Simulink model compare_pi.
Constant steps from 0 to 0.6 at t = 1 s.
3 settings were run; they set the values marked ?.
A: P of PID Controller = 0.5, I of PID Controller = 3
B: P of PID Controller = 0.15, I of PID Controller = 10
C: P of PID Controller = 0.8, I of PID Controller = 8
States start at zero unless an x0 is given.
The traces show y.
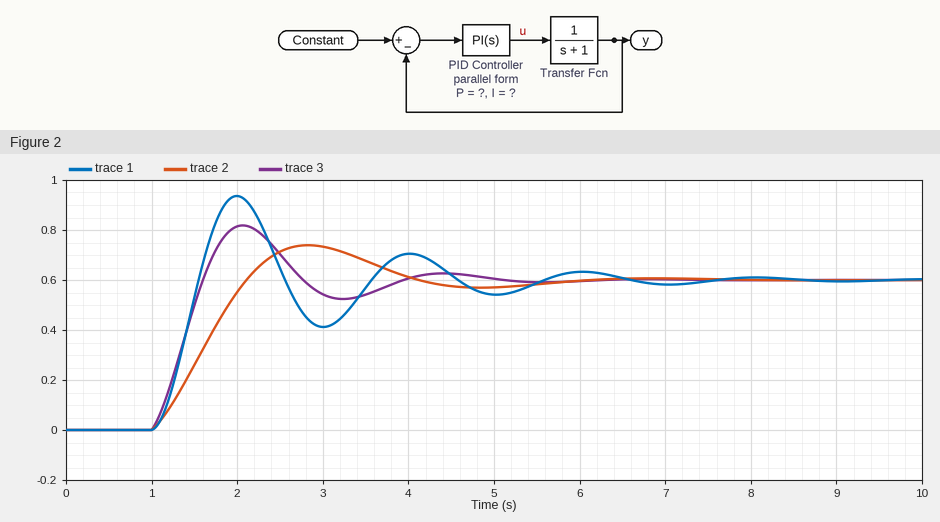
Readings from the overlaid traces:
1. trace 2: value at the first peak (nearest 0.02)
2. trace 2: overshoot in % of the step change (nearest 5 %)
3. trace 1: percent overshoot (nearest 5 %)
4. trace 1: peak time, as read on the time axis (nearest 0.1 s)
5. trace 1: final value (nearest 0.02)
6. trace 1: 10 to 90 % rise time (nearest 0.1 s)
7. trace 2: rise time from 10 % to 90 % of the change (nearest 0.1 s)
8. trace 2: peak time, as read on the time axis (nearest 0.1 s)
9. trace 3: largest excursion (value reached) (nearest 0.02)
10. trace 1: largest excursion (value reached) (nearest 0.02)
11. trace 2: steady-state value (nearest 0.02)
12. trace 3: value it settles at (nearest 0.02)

0.74
25 %
55 %
2.0 s
0.60
0.4 s
0.8 s
2.8 s
0.82
0.94
0.60
0.60
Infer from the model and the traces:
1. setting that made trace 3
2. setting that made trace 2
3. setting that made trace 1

C
A
B
